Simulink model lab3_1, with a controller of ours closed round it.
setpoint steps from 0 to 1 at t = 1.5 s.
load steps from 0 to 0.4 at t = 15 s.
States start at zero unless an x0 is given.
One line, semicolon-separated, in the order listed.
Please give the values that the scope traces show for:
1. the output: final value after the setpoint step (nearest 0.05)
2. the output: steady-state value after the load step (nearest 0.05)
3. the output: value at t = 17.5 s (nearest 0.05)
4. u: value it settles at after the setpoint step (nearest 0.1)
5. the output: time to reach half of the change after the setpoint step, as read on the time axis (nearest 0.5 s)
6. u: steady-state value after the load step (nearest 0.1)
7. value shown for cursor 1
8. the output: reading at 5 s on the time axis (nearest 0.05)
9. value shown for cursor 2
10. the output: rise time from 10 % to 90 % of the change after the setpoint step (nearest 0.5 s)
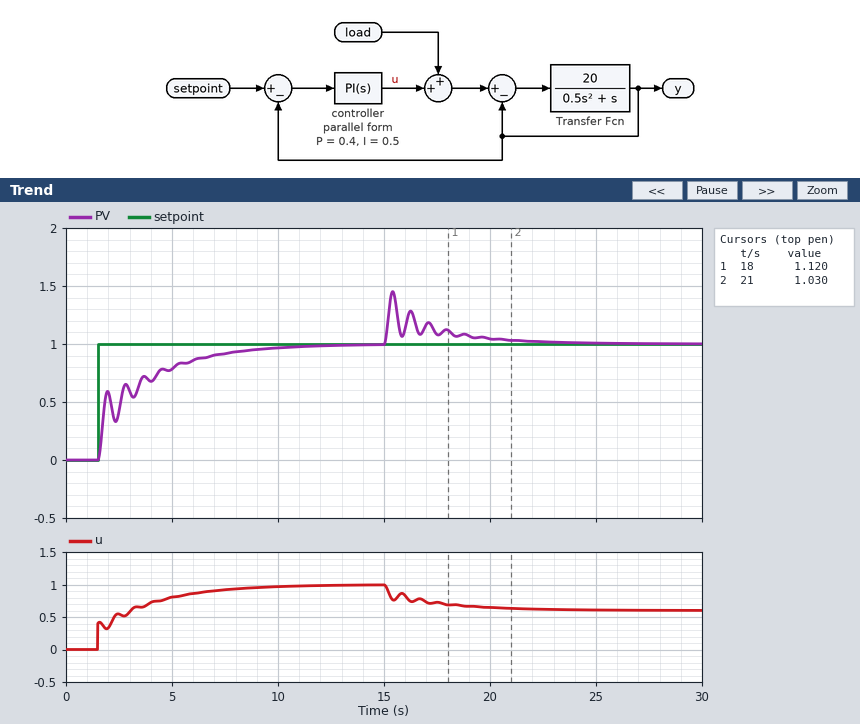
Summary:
1.00; 1.00; 1.10; 1.0; 2.0 s; 0.6; 1.120; 0.80; 1.030; 5.5 s
